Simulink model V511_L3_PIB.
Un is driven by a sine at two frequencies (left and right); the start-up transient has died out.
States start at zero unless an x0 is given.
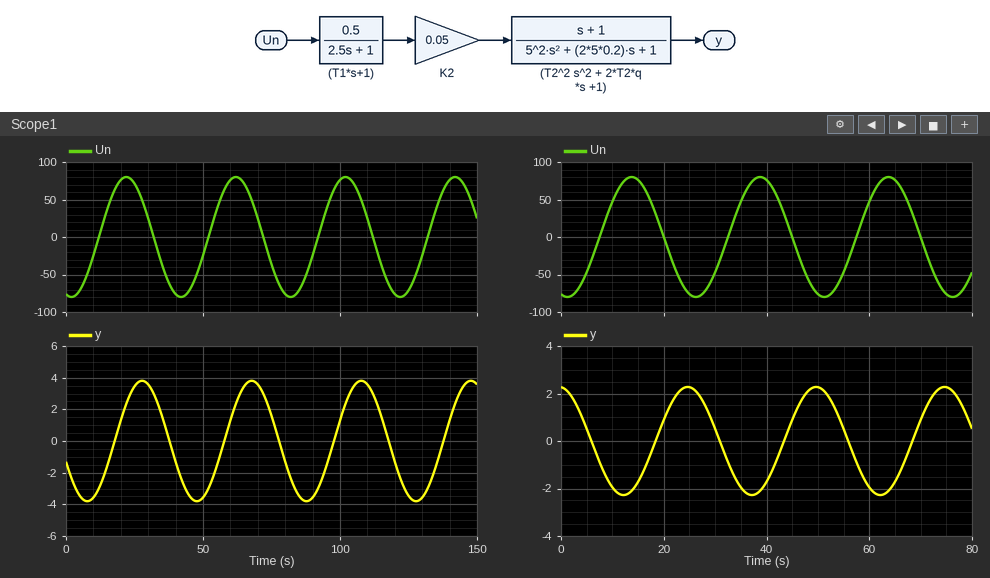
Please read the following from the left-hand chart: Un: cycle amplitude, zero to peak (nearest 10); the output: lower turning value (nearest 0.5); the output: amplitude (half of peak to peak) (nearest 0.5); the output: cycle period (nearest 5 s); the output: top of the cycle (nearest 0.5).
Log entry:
80
-4.0
4.0
40 s
4.0
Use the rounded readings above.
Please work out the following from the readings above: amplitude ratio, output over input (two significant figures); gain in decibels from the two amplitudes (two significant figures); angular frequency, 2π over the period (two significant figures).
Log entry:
0.050
-26 dB
0.16 rad/s
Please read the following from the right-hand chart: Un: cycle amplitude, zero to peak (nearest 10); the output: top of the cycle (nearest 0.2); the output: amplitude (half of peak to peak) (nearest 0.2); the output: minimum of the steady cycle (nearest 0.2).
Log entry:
80
2.2
2.2
-2.2
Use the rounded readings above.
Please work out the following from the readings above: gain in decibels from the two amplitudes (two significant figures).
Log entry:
-31 dB
